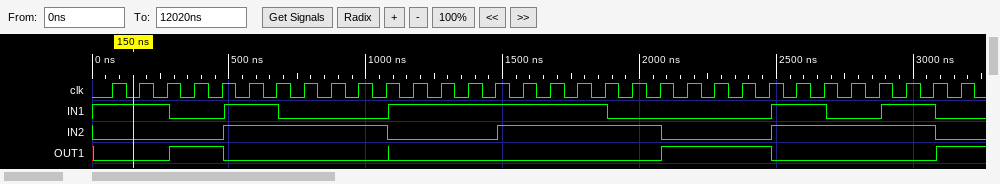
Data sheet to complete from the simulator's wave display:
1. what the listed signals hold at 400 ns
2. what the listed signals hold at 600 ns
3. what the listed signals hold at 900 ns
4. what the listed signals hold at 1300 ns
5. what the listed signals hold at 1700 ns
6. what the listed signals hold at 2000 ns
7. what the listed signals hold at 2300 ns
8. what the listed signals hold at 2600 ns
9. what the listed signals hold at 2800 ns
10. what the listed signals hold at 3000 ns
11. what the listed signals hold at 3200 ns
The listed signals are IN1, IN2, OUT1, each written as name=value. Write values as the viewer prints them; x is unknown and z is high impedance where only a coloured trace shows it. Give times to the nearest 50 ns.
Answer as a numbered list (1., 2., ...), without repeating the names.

1. IN1=0, IN2=0, OUT1=1
2. IN1=1, IN2=1, OUT1=0
3. IN1=0, IN2=1, OUT1=0
4. IN1=1, IN2=0, OUT1=0
5. IN1=1, IN2=1, OUT1=0
6. IN1=0, IN2=1, OUT1=0
7. IN1=0, IN2=0, OUT1=1
8. IN1=1, IN2=1, OUT1=0
9. IN1=0, IN2=1, OUT1=0
10. IN1=1, IN2=1, OUT1=0
11. IN1=0, IN2=0, OUT1=1
